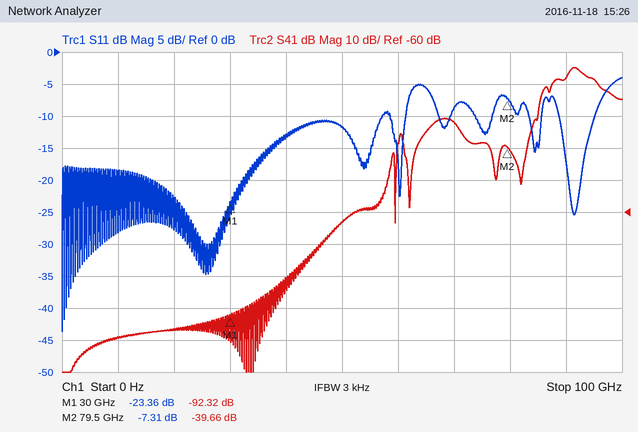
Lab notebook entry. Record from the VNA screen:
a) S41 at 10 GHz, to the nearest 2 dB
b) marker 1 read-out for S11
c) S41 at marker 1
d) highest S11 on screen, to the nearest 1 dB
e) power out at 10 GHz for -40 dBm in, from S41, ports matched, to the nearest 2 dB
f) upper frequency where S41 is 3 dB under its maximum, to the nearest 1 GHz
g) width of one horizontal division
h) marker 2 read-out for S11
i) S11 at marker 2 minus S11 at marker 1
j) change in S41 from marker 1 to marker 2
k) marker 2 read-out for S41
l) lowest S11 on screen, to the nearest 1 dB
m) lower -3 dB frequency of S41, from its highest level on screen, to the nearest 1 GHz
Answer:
-100 dB
-23.36 dB
-92.32 dB
-4 dB
-140 dBm
94 GHz
10 GHz
-7.31 dB
16.05 dB
52.66 dB
-39.66 dB
-44 dB
90 GHz
